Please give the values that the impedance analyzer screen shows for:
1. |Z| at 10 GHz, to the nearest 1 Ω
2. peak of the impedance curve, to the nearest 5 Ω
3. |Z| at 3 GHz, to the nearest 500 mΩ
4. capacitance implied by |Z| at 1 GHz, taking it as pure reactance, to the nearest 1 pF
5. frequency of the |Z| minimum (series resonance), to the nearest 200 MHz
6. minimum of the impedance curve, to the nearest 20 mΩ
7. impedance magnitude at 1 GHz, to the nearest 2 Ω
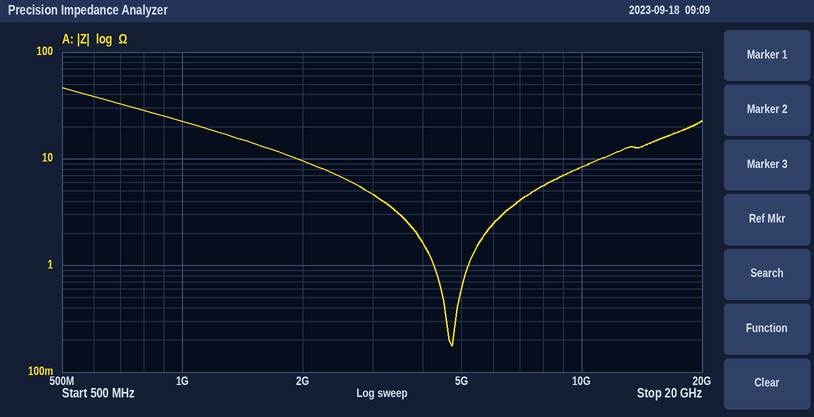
8 Ω
45 Ω
4.5 Ω
7 pF
4.8 GHz
180 mΩ
22 Ω
